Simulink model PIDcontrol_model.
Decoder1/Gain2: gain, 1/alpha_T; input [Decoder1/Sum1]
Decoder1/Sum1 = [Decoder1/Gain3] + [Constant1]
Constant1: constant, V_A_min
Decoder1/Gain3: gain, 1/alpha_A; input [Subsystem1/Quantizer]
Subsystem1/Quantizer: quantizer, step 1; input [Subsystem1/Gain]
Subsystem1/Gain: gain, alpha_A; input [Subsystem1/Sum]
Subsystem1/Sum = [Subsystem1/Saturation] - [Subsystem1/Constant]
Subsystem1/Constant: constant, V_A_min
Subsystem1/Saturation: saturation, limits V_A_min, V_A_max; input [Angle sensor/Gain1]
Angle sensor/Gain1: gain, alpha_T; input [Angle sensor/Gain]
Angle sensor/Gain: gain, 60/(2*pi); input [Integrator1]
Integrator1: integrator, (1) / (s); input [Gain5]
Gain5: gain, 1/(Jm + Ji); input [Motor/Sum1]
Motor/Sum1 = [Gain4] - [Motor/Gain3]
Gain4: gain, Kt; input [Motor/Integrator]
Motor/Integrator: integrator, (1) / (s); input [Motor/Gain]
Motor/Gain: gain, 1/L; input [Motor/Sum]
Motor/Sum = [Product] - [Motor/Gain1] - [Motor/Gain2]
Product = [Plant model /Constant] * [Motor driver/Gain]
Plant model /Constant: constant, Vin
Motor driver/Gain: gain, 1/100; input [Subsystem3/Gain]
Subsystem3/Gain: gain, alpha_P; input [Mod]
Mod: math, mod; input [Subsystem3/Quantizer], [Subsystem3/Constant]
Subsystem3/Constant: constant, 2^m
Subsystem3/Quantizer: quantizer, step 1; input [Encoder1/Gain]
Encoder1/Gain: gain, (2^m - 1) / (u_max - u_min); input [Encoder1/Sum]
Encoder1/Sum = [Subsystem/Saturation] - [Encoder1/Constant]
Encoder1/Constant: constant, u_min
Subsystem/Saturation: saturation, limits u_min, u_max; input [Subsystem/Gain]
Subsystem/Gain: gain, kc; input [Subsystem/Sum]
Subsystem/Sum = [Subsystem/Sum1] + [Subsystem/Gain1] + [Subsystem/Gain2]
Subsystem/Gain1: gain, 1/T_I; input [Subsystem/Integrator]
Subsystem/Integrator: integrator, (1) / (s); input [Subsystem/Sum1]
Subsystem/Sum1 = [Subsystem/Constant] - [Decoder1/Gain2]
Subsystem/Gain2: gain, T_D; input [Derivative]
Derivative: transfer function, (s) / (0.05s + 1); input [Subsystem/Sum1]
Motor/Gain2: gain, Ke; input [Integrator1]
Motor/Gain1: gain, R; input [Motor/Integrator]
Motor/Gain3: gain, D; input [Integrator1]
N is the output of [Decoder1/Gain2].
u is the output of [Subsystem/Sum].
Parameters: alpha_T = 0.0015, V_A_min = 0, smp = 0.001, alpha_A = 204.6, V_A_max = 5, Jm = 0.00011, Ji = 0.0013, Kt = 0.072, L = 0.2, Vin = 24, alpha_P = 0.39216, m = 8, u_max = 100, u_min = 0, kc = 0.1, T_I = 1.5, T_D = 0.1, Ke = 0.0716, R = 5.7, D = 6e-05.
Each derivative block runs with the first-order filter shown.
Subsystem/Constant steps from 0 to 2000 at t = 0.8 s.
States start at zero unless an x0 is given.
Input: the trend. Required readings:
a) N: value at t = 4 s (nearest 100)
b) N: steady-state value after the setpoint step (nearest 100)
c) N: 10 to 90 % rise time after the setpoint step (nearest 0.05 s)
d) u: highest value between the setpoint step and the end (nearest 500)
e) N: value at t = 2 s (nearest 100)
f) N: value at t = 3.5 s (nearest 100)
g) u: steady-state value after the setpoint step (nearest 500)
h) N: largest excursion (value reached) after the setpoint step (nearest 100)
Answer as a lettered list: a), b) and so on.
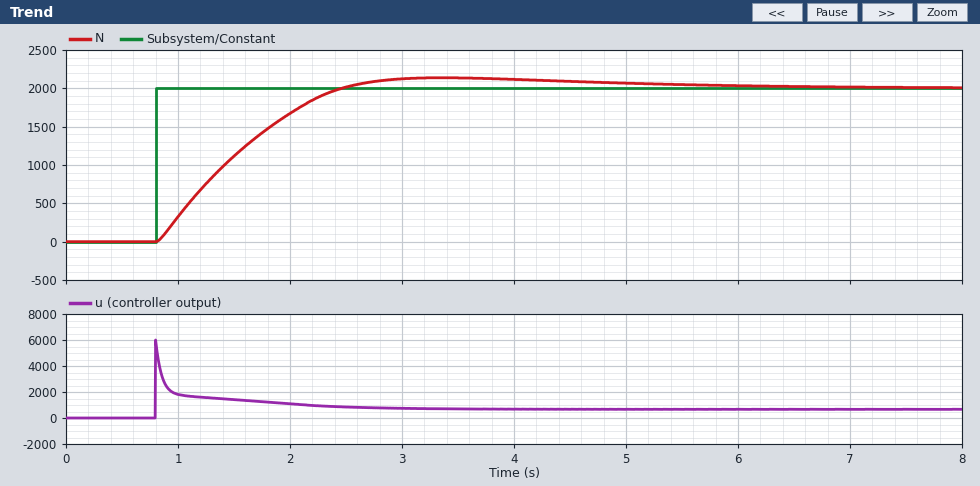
a) 2100
b) 2000
c) 1.20 s
d) 6000
e) 1700
f) 2100
g) 500
h) 2100
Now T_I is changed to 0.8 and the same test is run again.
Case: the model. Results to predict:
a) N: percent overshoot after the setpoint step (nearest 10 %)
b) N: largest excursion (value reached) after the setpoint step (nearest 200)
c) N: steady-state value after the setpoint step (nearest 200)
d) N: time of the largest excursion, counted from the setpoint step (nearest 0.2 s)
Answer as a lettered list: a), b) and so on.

a) 20 %
b) 2400
c) 2000
d) 2.6 s
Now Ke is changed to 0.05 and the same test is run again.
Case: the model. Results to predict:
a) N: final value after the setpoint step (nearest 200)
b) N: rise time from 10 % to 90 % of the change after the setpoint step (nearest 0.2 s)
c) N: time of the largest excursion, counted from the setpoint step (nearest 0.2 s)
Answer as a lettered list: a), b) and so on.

a) 2000
b) 1.0 s
c) 2.2 s
